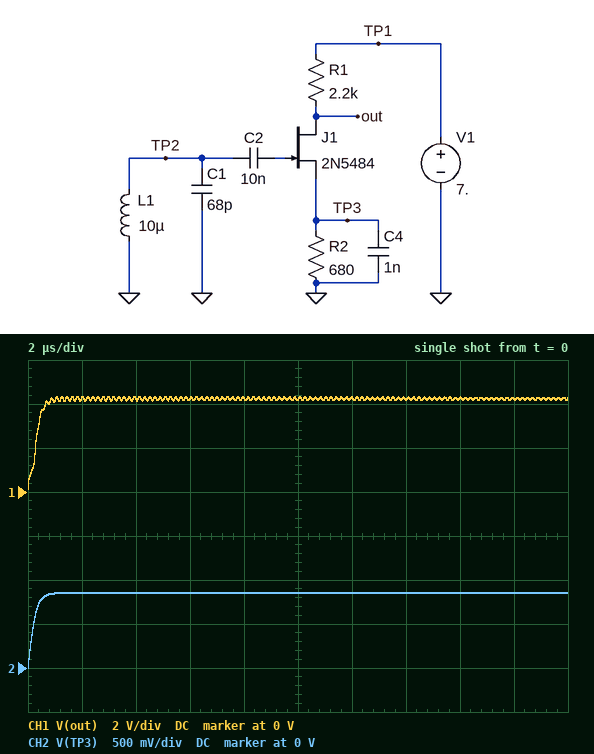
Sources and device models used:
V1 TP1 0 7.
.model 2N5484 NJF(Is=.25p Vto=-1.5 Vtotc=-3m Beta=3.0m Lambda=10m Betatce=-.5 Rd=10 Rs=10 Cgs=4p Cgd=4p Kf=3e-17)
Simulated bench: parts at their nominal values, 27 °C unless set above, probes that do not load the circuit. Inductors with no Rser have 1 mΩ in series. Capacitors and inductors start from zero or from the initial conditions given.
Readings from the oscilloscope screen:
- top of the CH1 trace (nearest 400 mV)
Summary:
4.4 V
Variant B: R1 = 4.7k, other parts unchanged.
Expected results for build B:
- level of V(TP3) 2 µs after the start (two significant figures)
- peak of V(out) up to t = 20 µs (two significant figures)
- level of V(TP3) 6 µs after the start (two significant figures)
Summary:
800 mV
1.3 V
820 mV
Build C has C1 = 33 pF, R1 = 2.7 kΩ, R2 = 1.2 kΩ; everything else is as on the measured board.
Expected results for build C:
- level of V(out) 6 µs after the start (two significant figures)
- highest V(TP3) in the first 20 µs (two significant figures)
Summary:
4.8 V
980 mV
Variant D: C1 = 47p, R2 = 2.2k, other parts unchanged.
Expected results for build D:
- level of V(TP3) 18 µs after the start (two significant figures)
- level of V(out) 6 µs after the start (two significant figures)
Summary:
1.1 V
5.9 V
